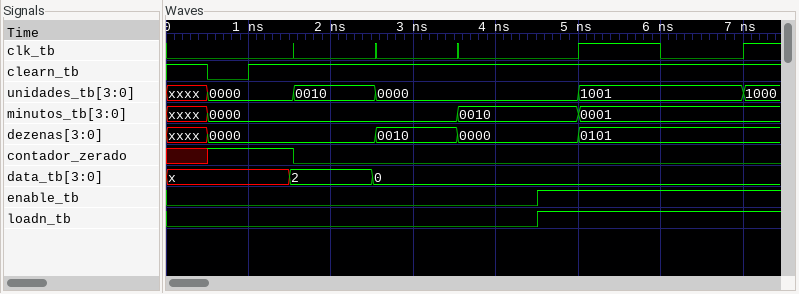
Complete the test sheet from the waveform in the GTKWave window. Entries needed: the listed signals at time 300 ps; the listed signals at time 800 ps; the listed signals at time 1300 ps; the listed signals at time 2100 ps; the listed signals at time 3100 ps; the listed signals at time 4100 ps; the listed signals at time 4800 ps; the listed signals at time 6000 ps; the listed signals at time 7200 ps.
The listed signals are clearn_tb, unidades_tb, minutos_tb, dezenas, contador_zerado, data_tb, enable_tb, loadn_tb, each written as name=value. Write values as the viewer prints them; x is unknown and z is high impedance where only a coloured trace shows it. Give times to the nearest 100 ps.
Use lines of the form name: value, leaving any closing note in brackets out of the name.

the listed signals at time 300 ps: clearn_tb=1, unidades_tb=xxxx, minutos_tb=xxxx, dezenas=xxxx, contador_zerado=x, data_tb=x, enable_tb=0, loadn_tb=0
the listed signals at time 800 ps: clearn_tb=0, unidades_tb=0000, minutos_tb=0000, dezenas=0000, contador_zerado=1, data_tb=x, enable_tb=0, loadn_tb=0
the listed signals at time 1300 ps: clearn_tb=1, unidades_tb=0000, minutos_tb=0000, dezenas=0000, contador_zerado=1, data_tb=x, enable_tb=0, loadn_tb=0
the listed signals at time 2100 ps: clearn_tb=1, unidades_tb=0010, minutos_tb=0000, dezenas=0000, contador_zerado=0, data_tb=2, enable_tb=0, loadn_tb=0
the listed signals at time 3100 ps: clearn_tb=1, unidades_tb=0000, minutos_tb=0000, dezenas=0010, contador_zerado=0, data_tb=0, enable_tb=0, loadn_tb=0
the listed signals at time 4100 ps: clearn_tb=1, unidades_tb=0000, minutos_tb=0010, dezenas=0000, contador_zerado=0, data_tb=0, enable_tb=0, loadn_tb=0
the listed signals at time 4800 ps: clearn_tb=1, unidades_tb=0000, minutos_tb=0010, dezenas=0000, contador_zerado=0, data_tb=0, enable_tb=1, loadn_tb=1
the listed signals at time 6000 ps: clearn_tb=1, unidades_tb=1001, minutos_tb=0001, dezenas=0101, contador_zerado=0, data_tb=0, enable_tb=1, loadn_tb=1
the listed signals at time 7200 ps: clearn_tb=1, unidades_tb=1000, minutos_tb=0001, dezenas=0101, contador_zerado=0, data_tb=0, enable_tb=1, loadn_tb=1
